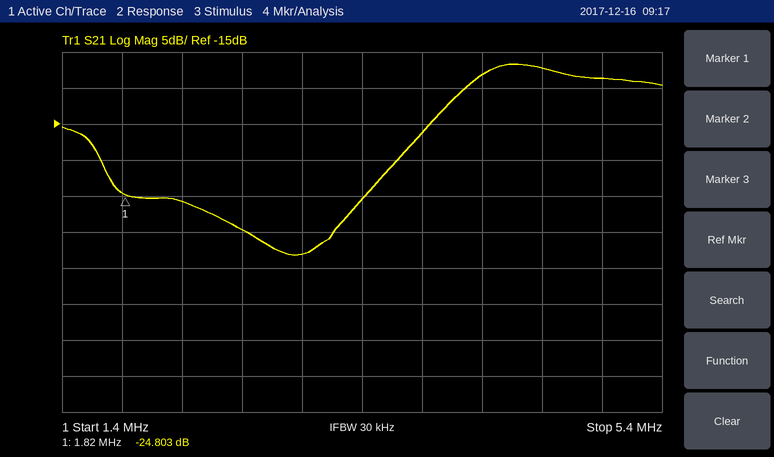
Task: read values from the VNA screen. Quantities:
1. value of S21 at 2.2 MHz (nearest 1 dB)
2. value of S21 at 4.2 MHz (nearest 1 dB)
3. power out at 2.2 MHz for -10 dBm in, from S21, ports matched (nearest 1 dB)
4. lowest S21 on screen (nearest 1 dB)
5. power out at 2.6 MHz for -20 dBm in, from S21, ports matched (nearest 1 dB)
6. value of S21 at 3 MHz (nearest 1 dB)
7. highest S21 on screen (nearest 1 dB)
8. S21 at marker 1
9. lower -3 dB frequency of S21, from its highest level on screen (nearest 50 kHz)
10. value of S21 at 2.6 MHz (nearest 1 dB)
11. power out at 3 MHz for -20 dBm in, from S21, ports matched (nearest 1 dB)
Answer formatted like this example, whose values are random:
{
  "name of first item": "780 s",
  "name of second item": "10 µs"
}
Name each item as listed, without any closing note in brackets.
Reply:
{
  "value of S21 at 2.2 MHz": "-26 dB",
  "value of S21 at 4.2 MHz": "-8 dB",
  "power out at 2.2 MHz for -10 dBm in, from S21, ports matched": "-36 dBm",
  "lowest S21 on screen": "-33 dB",
  "power out at 2.6 MHz for -20 dBm in, from S21, ports matched": "-50 dBm",
  "value of S21 at 3 MHz": "-33 dB",
  "highest S21 on screen": "-7 dB",
  "S21 at marker 1": "-24.803 dB",
  "lower -3 dB frequency of S21, from its highest level on screen": "4.10 MHz",
  "value of S21 at 2.6 MHz": "-30 dB",
  "power out at 3 MHz for -20 dBm in, from S21, ports matched": "-53 dBm"
}
